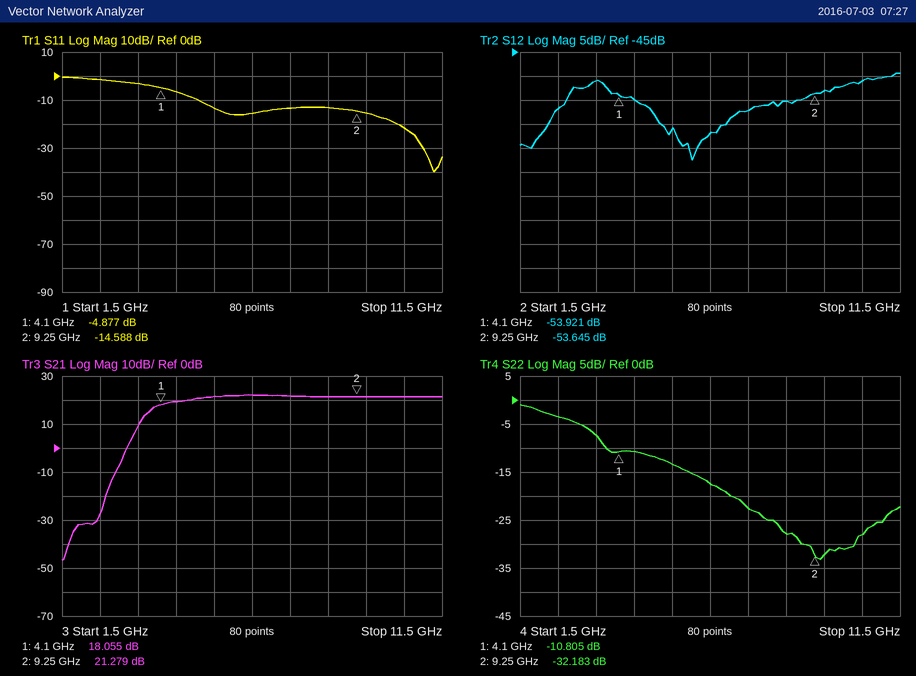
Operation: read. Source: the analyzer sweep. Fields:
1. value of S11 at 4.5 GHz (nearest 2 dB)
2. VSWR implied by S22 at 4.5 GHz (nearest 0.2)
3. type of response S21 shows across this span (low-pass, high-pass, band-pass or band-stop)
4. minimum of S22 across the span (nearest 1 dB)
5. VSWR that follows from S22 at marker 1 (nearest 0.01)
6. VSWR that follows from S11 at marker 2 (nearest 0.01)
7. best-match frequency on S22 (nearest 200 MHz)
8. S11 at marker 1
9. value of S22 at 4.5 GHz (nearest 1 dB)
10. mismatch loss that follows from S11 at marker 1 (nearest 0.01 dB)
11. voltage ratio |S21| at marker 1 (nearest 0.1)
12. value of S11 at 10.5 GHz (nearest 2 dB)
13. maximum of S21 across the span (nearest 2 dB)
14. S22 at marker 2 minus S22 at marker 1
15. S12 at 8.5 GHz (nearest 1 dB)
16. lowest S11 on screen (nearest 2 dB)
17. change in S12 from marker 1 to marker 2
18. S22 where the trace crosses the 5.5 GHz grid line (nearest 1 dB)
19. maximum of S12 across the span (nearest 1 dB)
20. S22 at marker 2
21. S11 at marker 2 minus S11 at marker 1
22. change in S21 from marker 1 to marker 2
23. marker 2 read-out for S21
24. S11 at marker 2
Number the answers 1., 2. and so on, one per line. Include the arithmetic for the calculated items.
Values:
1. -6 dB
2. |Γ| = 10^(-11/20) = 0.2818; VSWR = (1 + 0.2818)/(1 − 0.2818) ≈ 1.8
3. high-pass
4. -33 dB
5. (1 + 0.2882)/(1 − 0.2882) ≈ 1.81
6. (1 + 0.1865)/(1 − 0.1865) ≈ 1.46
7. 9.4 GHz
8. -4.877 dB
9. -11 dB
10. −10 log10(1 − 10^(-4.877/10)) ≈ 1.71 dB
11. 10^(18.055/20) ≈ 8.0
12. -22 dB
13. 22 dB
14. -32.183 − (-10.805) = -21.378 dB
15. -55 dB
16. -40 dB
17. -53.645 − (-53.921) = 0.276 dB
18. -13 dB
19. -49 dB
20. -32.183 dB
21. -14.588 − (-4.877) = -9.711 dB
22. 21.279 − (18.055) = 3.224 dB
23. 21.279 dB
24. -14.588 dB
